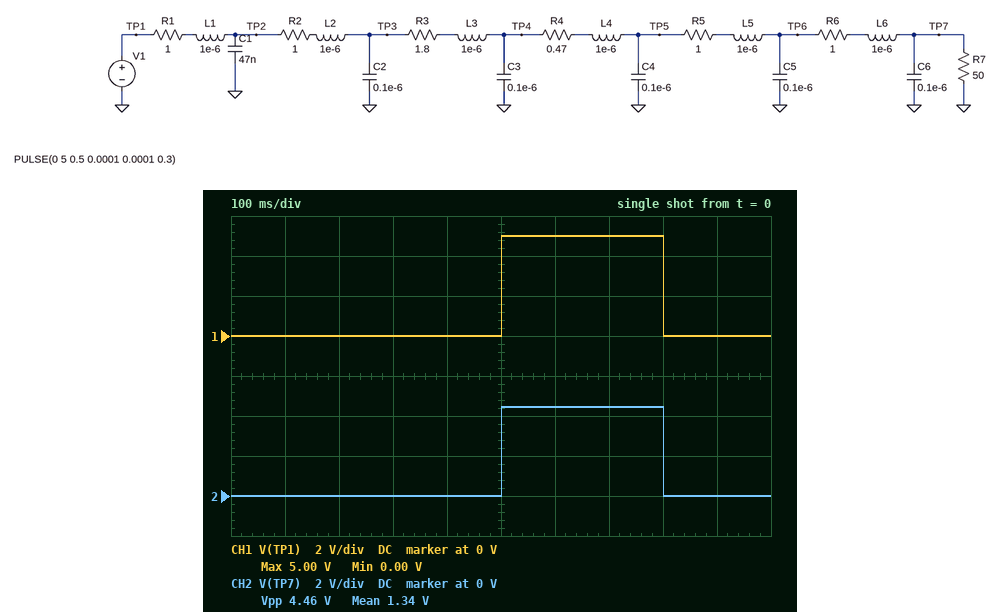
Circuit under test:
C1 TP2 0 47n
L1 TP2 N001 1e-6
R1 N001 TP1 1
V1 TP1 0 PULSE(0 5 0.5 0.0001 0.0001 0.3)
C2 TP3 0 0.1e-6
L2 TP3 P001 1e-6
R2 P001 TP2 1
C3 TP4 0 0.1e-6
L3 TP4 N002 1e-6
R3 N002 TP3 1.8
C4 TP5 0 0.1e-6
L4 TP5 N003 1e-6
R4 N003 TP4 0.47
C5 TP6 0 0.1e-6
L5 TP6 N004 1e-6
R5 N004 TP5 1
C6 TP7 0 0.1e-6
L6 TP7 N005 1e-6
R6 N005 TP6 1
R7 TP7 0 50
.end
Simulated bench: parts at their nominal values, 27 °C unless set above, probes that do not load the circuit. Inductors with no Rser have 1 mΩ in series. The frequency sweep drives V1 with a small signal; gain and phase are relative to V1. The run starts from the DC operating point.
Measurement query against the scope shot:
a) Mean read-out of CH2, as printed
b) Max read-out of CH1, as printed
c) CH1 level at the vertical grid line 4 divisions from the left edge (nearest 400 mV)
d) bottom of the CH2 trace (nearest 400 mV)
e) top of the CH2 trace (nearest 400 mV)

1.34 V
5.00 V
0 V
0 V
4.4 V
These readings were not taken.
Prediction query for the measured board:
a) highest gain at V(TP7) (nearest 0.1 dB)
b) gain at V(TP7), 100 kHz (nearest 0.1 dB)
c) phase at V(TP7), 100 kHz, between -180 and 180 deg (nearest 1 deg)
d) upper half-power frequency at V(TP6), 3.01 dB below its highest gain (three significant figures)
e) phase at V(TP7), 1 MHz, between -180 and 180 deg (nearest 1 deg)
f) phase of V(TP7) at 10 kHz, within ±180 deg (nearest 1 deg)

-0.9 dB
-1.4 dB
-84 deg
152 kHz
-90 deg
-8 deg
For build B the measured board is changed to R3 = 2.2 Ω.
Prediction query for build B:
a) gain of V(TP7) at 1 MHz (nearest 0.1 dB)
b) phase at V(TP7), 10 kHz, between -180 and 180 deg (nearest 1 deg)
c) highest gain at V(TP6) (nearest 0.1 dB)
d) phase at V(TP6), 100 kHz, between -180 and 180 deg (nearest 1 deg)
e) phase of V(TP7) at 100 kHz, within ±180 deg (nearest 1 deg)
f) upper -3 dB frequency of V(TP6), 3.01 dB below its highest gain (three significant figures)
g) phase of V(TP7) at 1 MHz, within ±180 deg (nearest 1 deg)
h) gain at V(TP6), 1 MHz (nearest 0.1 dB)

-27.9 dB
-8 deg
-0.9 dB
-81 deg
-85 deg
142 kHz
-86 deg
-18.3 dB
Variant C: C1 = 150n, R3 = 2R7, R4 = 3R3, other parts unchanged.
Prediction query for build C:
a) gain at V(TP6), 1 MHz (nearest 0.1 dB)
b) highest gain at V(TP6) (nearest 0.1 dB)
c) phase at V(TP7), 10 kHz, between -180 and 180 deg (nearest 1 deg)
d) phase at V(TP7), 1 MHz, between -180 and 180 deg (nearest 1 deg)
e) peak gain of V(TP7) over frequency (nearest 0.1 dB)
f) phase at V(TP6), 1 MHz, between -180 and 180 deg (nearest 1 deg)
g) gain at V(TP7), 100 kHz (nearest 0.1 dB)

-39.0 dB
-1.4 dB
-11 deg
-167 deg
-1.6 dB
-1 deg
-4.7 dB
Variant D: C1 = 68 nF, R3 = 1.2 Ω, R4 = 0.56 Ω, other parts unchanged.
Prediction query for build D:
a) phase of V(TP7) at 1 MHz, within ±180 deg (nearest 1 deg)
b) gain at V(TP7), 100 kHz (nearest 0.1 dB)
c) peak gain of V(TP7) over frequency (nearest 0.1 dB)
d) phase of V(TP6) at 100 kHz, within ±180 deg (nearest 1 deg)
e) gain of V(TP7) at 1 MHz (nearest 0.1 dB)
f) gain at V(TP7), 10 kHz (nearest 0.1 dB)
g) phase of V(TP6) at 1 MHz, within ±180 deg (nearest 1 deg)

-156 deg
-0.5 dB
-0.4 dB
-78 deg
-25.6 dB
-0.9 dB
10 deg
